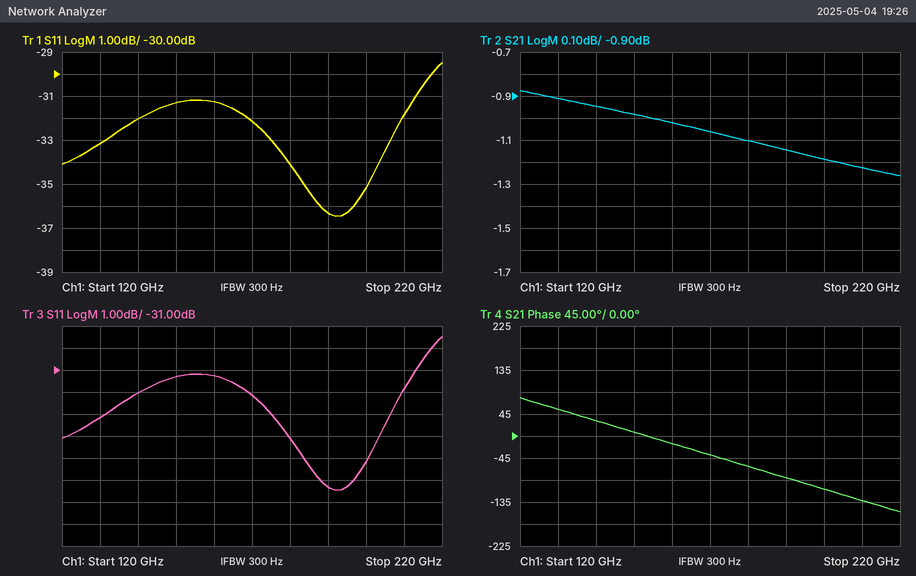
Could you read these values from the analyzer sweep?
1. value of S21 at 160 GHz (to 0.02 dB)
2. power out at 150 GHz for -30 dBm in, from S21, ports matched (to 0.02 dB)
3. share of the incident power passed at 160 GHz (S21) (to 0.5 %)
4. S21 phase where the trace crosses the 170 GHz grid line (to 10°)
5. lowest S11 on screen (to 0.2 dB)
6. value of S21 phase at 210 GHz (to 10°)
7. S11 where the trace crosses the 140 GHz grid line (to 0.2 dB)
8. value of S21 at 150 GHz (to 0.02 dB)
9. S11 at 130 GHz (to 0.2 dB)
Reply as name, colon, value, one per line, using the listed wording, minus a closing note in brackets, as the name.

value of S21 at 160 GHz: -1.02 dB
power out at 150 GHz for -30 dBm in, from S21, ports matched: -30.98 dBm
share of the incident power passed at 160 GHz (S21): 79.0 %
S21 phase where the trace crosses the 170 GHz grid line: -40°
lowest S11 on screen: -36.4 dB
value of S21 phase at 210 GHz: -130°
S11 where the trace crosses the 140 GHz grid line: -32.0 dB
value of S21 at 150 GHz: -0.98 dB
S11 at 130 GHz: -33.2 dB
